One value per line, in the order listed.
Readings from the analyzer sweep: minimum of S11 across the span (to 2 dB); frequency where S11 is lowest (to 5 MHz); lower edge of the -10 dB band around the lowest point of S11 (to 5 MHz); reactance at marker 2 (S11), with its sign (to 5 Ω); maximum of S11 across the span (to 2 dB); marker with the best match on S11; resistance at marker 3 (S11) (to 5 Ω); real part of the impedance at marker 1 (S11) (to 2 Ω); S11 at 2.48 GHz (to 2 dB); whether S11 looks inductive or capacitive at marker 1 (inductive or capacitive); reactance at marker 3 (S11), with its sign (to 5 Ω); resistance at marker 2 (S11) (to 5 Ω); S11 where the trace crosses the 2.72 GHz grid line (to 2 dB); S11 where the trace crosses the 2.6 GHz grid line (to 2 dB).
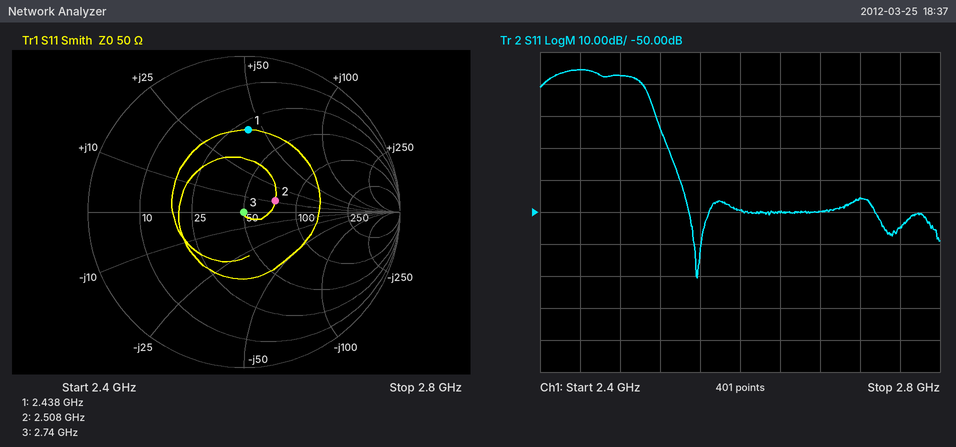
-70 dB
2.555 GHz
2.500 GHz
+10 Ω
-6 dB
marker 3
50 Ω
30 Ω
-8 dB
inductive
0 Ω
75 Ω
-46 dB
-50 dB
